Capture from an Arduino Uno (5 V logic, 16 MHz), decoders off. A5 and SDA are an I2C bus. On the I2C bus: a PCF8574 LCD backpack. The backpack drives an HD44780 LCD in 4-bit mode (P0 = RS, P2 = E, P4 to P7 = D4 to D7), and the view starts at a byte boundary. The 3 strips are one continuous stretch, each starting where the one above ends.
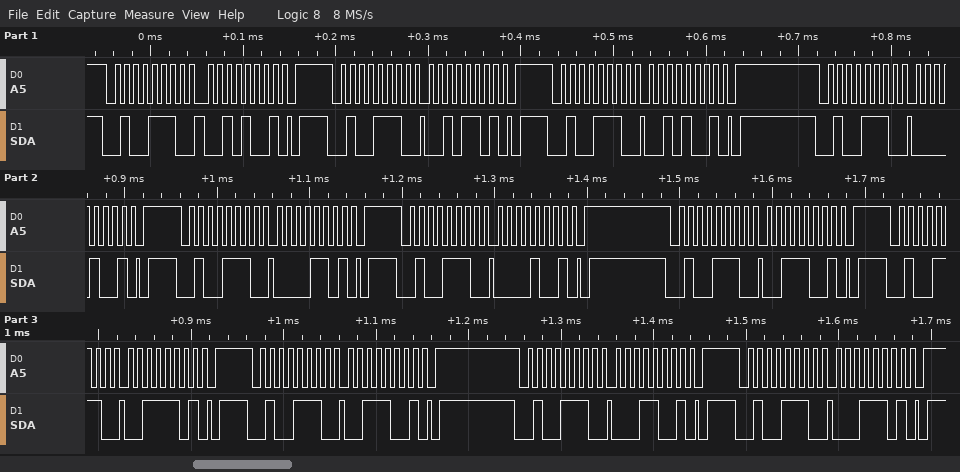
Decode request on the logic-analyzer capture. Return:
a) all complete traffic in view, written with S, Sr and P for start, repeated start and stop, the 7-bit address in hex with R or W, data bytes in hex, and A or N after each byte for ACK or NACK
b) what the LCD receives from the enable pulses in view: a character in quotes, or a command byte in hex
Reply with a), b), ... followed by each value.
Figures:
a) S 27W A 29 A P S 27W A 2D A P S 27W A 29 A P S 27W A 09 A P S 27W A 0D A P S 27W A 09 A P S 27W A 39 A P S 27W A 3D A P S 27W A 39 A P S 27W A 19 A P S 27W A 1D A P
b) ' '
